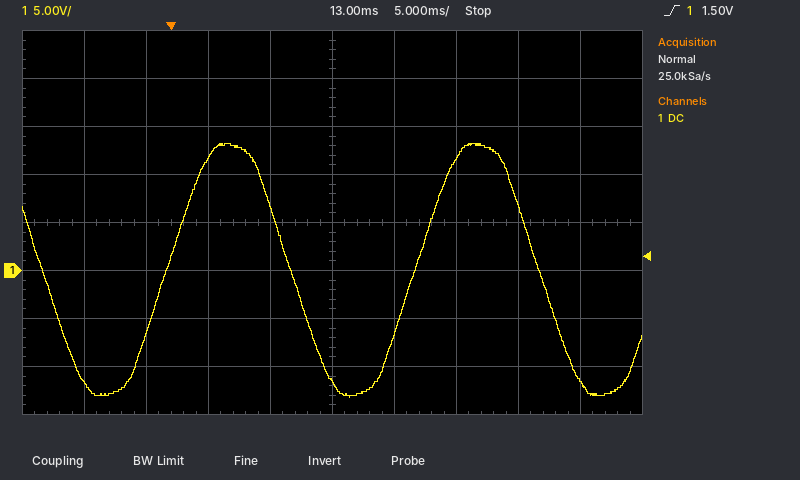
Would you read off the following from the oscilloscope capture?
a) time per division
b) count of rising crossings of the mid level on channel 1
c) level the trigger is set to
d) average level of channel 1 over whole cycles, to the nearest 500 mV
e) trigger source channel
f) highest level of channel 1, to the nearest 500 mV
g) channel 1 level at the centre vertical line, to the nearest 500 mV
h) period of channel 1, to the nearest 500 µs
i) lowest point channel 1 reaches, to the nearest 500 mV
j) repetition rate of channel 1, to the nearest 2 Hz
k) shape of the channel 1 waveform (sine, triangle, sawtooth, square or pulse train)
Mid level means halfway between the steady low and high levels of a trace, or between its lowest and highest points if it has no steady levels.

5 ms
2
1.50 V
0.0 V
channel 1
13.0 V
-11.5 V
20.0 ms
-13.0 V
50 Hz
sine
